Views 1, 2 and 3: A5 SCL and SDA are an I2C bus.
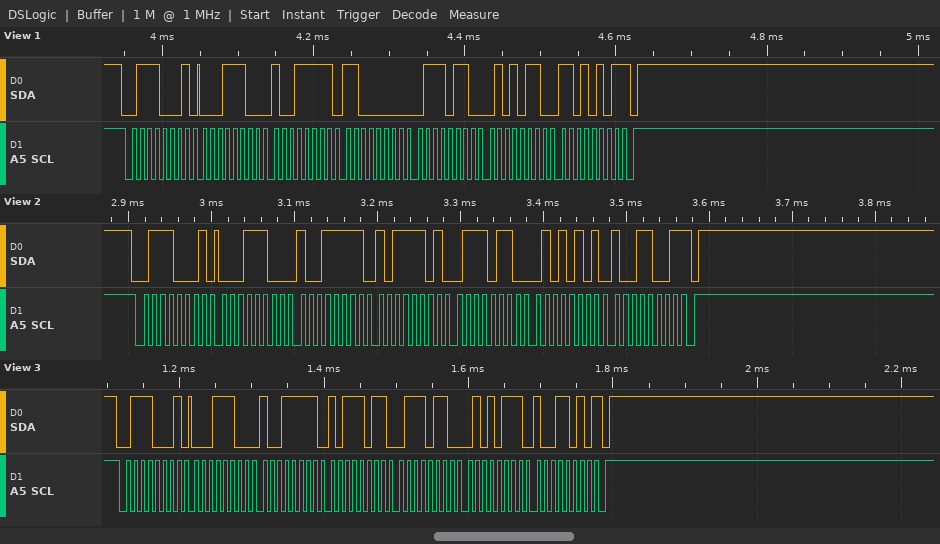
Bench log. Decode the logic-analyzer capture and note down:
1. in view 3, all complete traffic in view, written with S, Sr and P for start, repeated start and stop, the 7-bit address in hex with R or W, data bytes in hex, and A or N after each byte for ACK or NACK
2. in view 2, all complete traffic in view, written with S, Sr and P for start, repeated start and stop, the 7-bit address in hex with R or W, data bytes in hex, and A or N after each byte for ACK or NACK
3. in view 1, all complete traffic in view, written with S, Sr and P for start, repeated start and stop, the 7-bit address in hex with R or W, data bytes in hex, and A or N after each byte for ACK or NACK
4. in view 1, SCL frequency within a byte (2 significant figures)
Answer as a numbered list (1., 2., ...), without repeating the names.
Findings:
1. S 38R A 1C A 9F A BB A 76 A 57 A 9A N P
2. S 38R A 1C A 9F A BD A 76 A 55 A 99 N P
3. S 38R A 1C A 9F A C0 A 76 A 56 A D5 N P
4. 100 kHz
